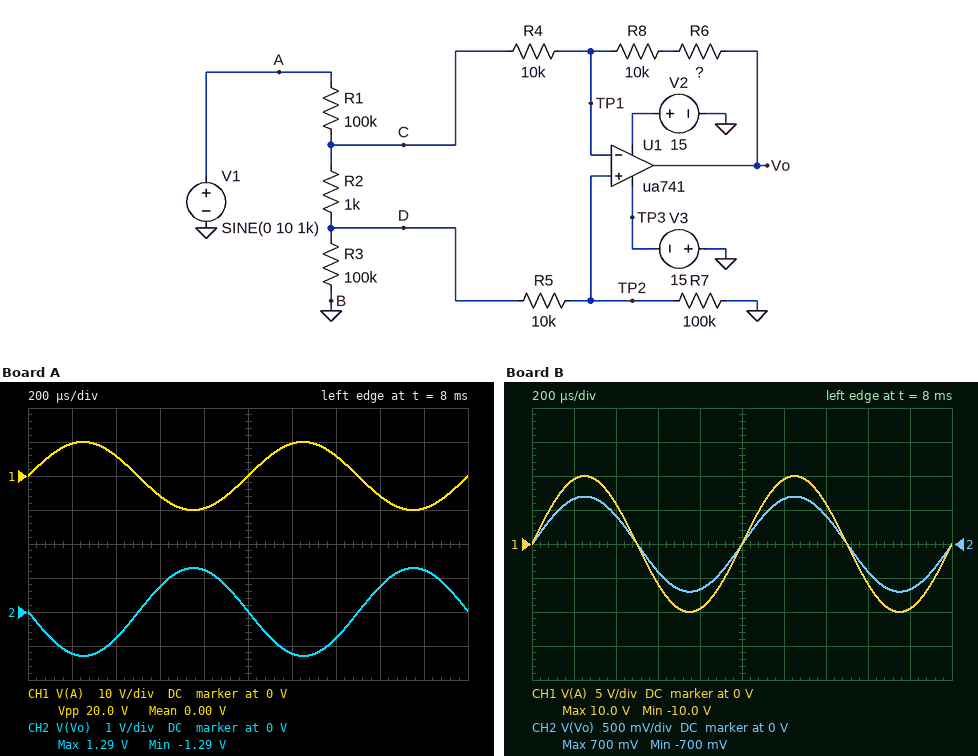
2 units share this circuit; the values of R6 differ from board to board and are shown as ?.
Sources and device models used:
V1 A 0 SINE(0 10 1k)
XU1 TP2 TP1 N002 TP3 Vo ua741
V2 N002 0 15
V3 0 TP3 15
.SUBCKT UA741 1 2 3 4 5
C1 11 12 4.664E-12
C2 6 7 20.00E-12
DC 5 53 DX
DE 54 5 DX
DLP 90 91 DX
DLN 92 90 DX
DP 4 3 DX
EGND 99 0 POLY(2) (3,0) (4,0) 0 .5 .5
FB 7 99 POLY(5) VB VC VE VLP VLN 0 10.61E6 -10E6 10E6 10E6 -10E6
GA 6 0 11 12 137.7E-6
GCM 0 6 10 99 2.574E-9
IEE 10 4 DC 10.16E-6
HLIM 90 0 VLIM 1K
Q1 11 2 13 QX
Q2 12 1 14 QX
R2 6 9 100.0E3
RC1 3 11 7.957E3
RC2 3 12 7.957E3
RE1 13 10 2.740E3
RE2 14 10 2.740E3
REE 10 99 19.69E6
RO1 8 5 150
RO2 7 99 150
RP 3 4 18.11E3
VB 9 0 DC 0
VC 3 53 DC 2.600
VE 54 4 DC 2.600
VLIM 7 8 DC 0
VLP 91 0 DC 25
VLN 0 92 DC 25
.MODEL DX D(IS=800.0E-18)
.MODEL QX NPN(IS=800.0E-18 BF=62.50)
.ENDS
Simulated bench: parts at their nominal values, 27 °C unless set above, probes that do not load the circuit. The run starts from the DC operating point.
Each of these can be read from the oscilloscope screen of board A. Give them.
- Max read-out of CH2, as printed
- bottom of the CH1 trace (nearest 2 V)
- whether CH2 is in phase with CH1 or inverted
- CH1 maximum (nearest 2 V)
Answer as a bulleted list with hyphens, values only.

- 1.29 V
- -10 V
- inverted
- 10 V
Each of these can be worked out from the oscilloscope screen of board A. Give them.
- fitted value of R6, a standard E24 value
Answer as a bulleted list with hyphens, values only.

- 120 kΩ
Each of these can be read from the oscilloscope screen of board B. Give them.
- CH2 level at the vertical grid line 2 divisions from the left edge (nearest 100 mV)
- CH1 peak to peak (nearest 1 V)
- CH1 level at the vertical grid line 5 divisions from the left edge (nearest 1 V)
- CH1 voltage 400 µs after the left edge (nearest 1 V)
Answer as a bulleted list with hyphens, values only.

- 400 mV
- 20 V
- 0 V
- 6 V
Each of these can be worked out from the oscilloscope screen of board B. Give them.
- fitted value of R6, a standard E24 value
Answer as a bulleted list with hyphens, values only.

- 47 kΩ
